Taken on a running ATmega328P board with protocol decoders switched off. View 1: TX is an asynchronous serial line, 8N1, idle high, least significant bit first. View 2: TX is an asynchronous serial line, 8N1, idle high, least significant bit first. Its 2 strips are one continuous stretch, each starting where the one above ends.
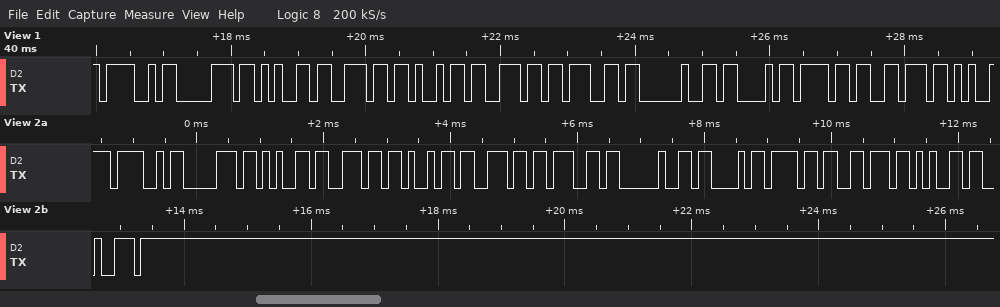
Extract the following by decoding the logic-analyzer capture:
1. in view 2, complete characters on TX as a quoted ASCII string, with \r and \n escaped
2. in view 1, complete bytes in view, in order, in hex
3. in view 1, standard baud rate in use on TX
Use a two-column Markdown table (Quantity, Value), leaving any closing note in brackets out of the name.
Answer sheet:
| Quantity | Value |
|---|---|
| in view 2, complete characters on TX as a quoted ASCII string, with \r and \n escaped | "Opening Cover" |
| in view 1, complete bytes in view, in order, in hex | 0x4F 0x70 0x65 0x6E 0x69 0x6E 0x67 0x20 0x43 0x6F 0x76 |
| in view 1, standard baud rate in use on TX | 9600 baud |
